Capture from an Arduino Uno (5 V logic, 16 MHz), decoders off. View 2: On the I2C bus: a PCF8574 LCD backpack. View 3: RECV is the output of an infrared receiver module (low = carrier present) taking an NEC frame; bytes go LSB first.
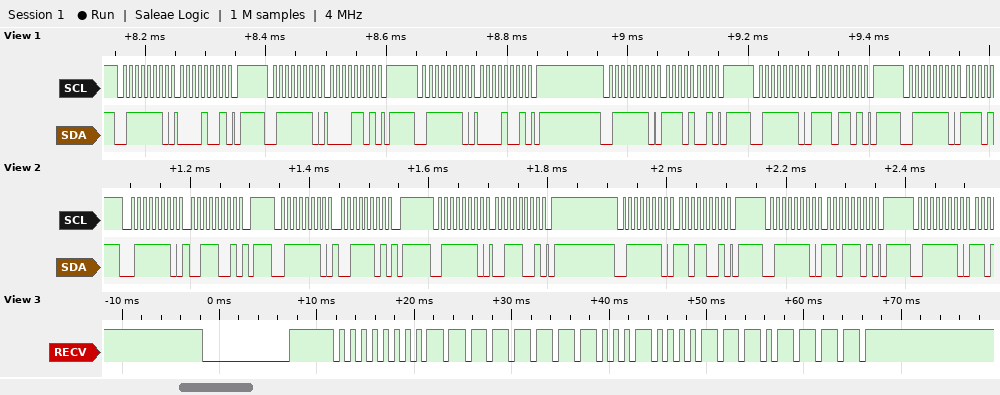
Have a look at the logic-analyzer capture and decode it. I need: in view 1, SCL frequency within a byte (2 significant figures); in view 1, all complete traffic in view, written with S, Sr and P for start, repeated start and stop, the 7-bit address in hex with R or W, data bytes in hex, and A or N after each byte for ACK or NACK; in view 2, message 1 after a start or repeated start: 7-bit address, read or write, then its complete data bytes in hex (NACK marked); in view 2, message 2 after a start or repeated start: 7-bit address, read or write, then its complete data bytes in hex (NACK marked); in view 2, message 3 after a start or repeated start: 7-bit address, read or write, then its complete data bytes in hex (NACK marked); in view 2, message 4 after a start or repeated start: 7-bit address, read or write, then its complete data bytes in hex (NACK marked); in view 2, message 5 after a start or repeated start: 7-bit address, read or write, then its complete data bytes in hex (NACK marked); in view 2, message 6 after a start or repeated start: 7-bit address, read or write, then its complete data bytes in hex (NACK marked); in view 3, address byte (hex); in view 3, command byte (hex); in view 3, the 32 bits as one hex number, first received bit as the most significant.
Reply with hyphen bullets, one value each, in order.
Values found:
- 100 kHz
- S 3FW A 09 A P S 3FW A 0D A P S 3FW A 09 A P S 3FW A E9 A P S 3FW A ED A P S 3FW A
- 0x3F write: 39
- 0x3F write: 3D
- 0x3F write: 39
- 0x3F write: D9
- 0x3F write: DD
- 0x3F write
- 0x00
- 0x08
- 0x00FF10EF
